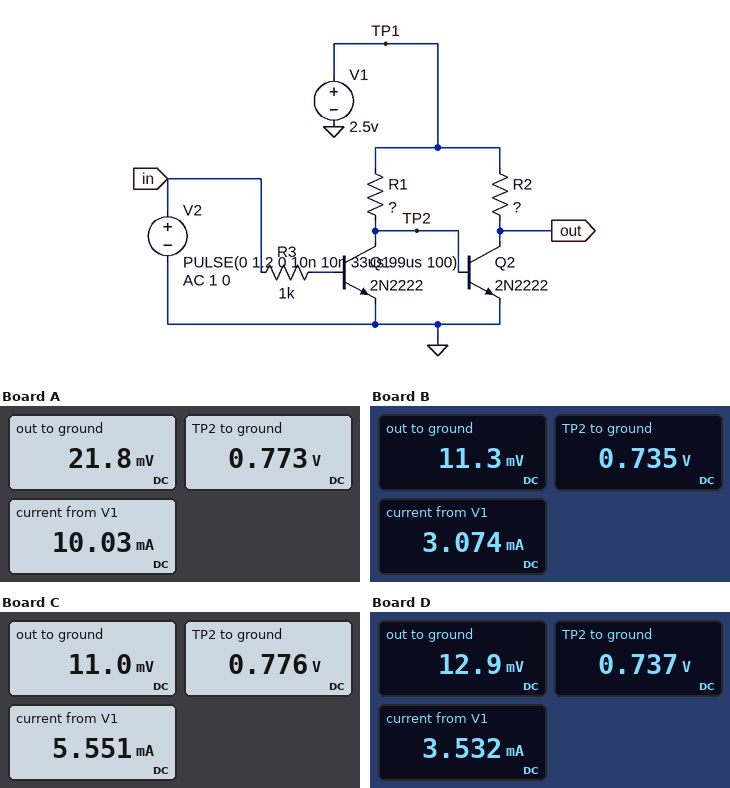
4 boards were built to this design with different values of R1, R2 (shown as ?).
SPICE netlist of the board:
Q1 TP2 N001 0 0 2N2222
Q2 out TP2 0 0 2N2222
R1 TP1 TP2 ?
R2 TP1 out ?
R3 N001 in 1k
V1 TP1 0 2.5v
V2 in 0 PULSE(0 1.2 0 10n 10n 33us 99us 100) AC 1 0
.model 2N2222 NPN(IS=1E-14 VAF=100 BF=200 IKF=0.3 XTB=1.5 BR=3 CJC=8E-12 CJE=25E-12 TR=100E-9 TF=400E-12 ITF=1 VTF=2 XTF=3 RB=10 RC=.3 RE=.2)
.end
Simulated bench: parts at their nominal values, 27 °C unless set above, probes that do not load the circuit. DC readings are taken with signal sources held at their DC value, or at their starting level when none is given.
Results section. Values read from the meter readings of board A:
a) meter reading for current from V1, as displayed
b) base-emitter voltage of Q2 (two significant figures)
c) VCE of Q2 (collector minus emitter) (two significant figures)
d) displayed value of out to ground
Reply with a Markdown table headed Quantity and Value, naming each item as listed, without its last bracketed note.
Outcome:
| Quantity | Value |
|---|---|
| meter reading for current from V1, as displayed | 10.03 mA |
| base-emitter voltage of Q2 | 770 mV |
| VCE of Q2 (collector minus emitter) | 22 mV |
| displayed value of out to ground | 21.8 mV |
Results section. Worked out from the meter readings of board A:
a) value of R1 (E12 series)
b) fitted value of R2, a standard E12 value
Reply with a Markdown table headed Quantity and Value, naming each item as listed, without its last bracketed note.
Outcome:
| Quantity | Value |
|---|---|
| value of R1 | 470 Ω |
| fitted value of R2, a standard E12 value | 390 Ω |
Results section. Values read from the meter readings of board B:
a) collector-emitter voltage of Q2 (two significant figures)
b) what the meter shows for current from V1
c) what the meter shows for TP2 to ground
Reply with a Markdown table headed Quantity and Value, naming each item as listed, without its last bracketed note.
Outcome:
| Quantity | Value |
|---|---|
| collector-emitter voltage of Q2 | 11 mV |
| what the meter shows for current from V1 | 3.074 mA |
| what the meter shows for TP2 to ground | 0.735 V |
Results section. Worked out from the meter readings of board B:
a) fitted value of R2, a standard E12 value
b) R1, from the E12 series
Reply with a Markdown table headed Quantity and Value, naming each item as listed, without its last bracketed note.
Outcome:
| Quantity | Value |
|---|---|
| fitted value of R2, a standard E12 value | 2.7 kΩ |
| R1, from the E12 series | 820 Ω |
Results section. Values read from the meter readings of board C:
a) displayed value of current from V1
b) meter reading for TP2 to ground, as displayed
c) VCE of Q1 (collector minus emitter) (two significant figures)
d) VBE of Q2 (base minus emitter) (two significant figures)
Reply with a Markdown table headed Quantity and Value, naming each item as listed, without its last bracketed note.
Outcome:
| Quantity | Value |
|---|---|
| displayed value of current from V1 | 5.551 mA |
| meter reading for TP2 to ground, as displayed | 0.776 V |
| VCE of Q1 (collector minus emitter) | 780 mV |
| VBE of Q2 (base minus emitter) | 780 mV |
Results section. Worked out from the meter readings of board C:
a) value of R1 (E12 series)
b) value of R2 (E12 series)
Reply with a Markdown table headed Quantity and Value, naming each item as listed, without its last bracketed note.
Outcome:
| Quantity | Value |
|---|---|
| value of R1 | 390 Ω |
| value of R2 | 2.2 kΩ |
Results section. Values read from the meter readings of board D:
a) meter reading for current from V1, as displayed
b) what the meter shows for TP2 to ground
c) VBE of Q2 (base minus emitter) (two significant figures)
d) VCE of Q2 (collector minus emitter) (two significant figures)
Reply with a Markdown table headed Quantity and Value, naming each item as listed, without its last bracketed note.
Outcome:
| Quantity | Value |
|---|---|
| meter reading for current from V1, as displayed | 3.532 mA |
| what the meter shows for TP2 to ground | 0.737 V |
| VBE of Q2 (base minus emitter) | 740 mV |
| VCE of Q2 (collector minus emitter) | 13 mV |
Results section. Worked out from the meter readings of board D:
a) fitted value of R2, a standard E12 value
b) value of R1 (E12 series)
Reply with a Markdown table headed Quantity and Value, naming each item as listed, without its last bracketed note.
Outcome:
| Quantity | Value |
|---|---|
| fitted value of R2, a standard E12 value | 1.8 kΩ |
| value of R1 | 820 Ω |
